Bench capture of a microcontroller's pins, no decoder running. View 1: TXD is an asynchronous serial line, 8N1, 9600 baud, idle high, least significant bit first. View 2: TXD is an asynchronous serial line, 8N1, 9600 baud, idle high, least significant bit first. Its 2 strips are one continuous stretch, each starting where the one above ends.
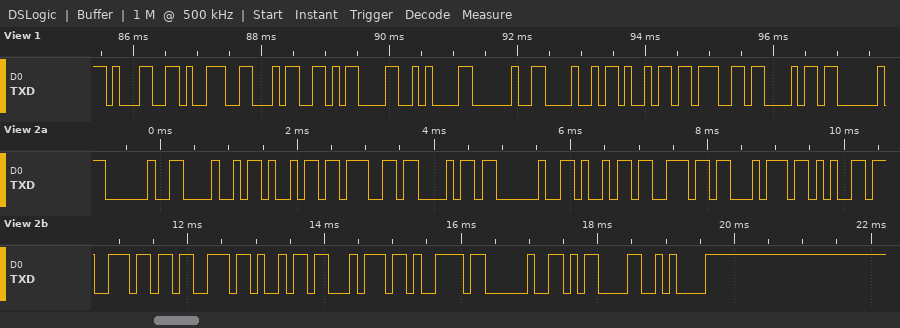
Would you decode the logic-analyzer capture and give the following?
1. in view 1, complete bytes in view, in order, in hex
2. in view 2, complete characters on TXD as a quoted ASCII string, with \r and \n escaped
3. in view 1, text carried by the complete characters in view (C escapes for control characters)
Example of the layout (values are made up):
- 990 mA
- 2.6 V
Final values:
- 31 39 34 0D 0A 20 48 69 67 68
- " High intensity \r\n"
- "194\r\n High"
